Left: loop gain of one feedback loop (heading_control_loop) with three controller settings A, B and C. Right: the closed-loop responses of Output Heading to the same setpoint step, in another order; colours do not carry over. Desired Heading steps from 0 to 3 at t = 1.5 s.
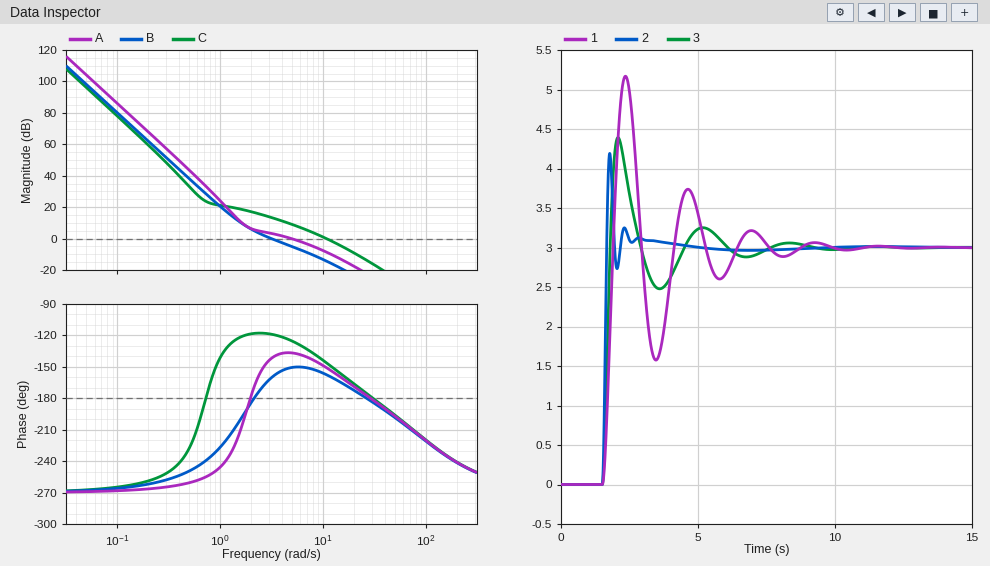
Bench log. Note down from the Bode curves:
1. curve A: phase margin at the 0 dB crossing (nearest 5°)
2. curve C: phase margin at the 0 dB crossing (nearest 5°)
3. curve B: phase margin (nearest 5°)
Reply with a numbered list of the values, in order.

1. 45°
2. 35°
3. 20°
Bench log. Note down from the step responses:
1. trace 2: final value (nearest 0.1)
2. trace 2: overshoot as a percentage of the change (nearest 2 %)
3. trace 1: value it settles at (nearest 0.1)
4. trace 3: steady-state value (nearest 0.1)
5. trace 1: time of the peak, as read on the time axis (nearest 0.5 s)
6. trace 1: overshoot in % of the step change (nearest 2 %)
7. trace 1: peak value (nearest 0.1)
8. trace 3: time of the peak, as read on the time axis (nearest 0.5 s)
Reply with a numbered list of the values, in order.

1. 3.0
2. 40 %
3. 3.0
4. 3.0
5. 2.5 s
6. 72 %
7. 5.2
8. 2.0 s
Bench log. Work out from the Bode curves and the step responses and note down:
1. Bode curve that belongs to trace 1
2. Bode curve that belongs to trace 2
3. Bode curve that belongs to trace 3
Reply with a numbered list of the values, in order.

1. B
2. C
3. A
